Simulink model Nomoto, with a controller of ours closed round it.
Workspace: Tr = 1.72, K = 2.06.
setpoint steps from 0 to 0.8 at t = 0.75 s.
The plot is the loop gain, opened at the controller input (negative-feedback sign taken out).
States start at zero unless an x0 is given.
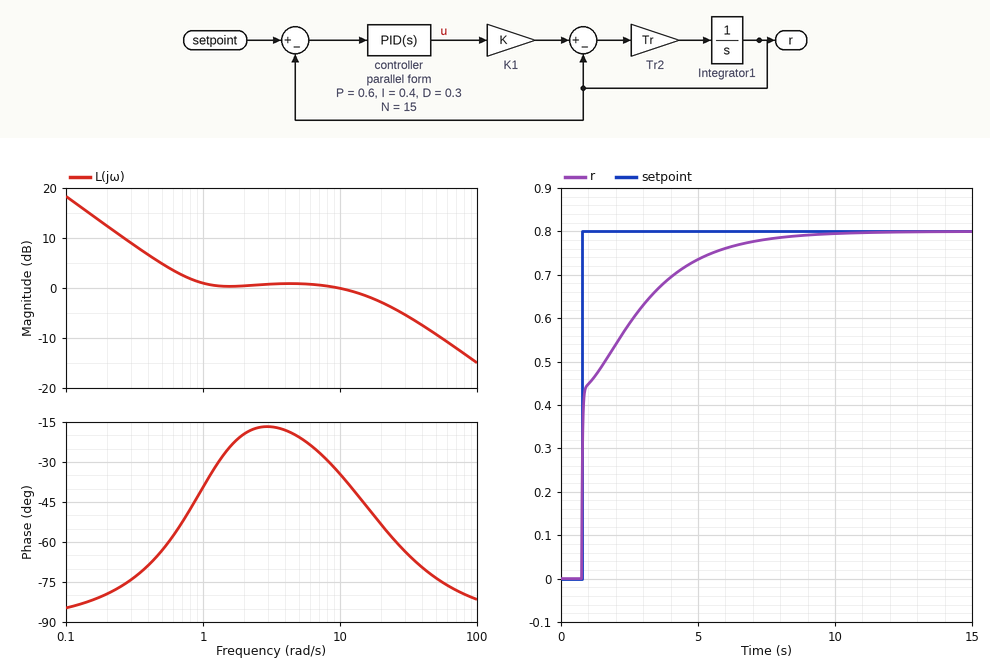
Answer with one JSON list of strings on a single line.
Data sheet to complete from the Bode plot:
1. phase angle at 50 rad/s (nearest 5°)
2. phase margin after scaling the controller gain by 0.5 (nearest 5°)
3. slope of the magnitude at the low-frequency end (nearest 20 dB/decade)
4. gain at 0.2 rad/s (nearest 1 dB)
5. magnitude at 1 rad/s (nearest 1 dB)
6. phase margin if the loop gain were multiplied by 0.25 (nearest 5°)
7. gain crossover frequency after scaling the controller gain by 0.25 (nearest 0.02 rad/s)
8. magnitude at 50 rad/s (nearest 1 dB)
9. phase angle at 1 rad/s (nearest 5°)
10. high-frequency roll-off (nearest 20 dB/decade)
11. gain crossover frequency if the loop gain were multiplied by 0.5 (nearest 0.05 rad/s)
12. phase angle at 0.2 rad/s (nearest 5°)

["-75°", "115°", "-20 dB/decade", "12 dB", "1 dB", "100°", "0.20 rad/s", "-9 dB", "-40°", "-20 dB/decade", "0.45 rad/s", "-80°"]
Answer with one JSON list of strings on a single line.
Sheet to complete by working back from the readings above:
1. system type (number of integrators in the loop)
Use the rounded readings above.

["1"]
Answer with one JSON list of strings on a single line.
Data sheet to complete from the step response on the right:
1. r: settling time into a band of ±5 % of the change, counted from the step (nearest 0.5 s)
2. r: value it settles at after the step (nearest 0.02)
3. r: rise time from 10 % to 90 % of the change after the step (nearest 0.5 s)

["5.0 s", "0.80", "4.0 s"]
